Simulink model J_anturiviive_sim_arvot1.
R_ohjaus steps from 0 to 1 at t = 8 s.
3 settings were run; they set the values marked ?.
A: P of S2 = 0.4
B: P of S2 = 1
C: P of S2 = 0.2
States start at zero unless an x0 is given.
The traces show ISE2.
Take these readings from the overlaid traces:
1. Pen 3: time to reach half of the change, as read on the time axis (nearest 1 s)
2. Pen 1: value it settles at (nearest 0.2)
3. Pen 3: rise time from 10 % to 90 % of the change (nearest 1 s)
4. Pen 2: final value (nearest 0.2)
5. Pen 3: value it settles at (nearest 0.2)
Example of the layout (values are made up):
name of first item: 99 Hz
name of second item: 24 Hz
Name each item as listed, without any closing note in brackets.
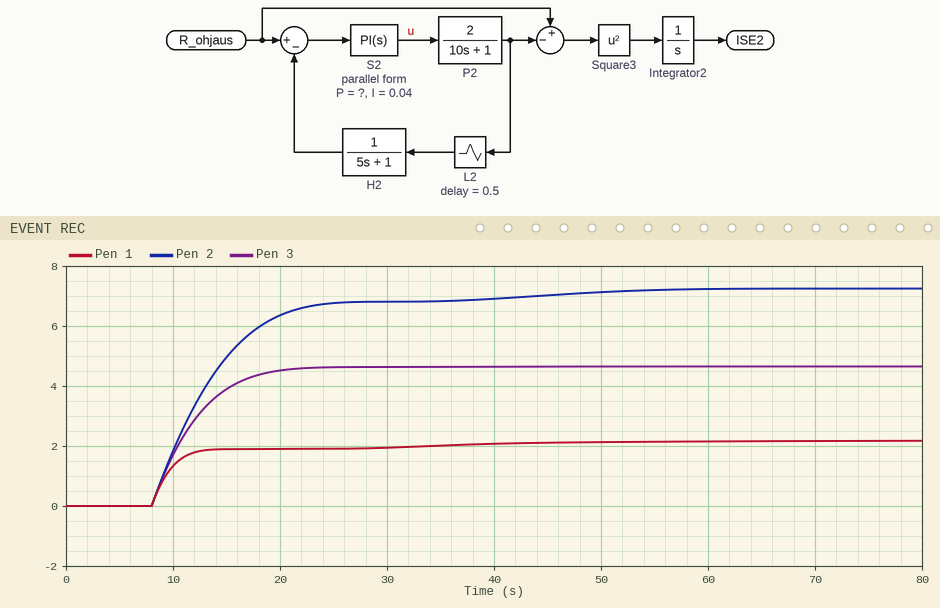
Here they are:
Pen 3: time to reach half of the change, as read on the time axis: 11 s
Pen 1: value it settles at: 2.2
Pen 3: rise time from 10 % to 90 % of the change: 8 s
Pen 2: final value: 7.2
Pen 3: value it settles at: 4.6
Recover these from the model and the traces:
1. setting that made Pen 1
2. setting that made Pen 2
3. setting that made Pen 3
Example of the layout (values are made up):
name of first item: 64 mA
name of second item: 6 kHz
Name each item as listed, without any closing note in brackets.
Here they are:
setting that made Pen 1: B
setting that made Pen 2: C
setting that made Pen 3: A
